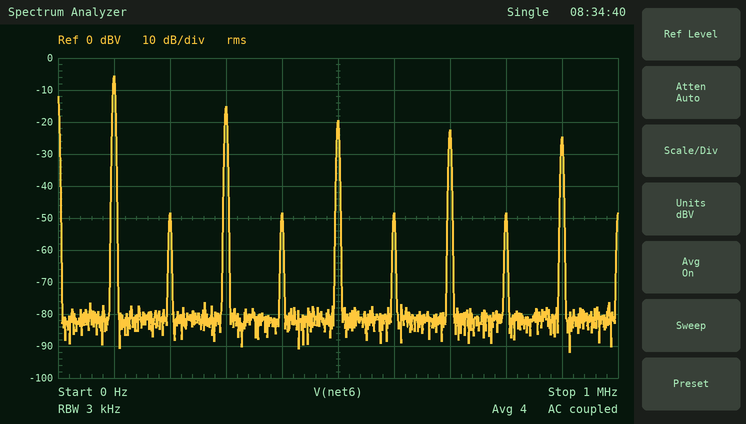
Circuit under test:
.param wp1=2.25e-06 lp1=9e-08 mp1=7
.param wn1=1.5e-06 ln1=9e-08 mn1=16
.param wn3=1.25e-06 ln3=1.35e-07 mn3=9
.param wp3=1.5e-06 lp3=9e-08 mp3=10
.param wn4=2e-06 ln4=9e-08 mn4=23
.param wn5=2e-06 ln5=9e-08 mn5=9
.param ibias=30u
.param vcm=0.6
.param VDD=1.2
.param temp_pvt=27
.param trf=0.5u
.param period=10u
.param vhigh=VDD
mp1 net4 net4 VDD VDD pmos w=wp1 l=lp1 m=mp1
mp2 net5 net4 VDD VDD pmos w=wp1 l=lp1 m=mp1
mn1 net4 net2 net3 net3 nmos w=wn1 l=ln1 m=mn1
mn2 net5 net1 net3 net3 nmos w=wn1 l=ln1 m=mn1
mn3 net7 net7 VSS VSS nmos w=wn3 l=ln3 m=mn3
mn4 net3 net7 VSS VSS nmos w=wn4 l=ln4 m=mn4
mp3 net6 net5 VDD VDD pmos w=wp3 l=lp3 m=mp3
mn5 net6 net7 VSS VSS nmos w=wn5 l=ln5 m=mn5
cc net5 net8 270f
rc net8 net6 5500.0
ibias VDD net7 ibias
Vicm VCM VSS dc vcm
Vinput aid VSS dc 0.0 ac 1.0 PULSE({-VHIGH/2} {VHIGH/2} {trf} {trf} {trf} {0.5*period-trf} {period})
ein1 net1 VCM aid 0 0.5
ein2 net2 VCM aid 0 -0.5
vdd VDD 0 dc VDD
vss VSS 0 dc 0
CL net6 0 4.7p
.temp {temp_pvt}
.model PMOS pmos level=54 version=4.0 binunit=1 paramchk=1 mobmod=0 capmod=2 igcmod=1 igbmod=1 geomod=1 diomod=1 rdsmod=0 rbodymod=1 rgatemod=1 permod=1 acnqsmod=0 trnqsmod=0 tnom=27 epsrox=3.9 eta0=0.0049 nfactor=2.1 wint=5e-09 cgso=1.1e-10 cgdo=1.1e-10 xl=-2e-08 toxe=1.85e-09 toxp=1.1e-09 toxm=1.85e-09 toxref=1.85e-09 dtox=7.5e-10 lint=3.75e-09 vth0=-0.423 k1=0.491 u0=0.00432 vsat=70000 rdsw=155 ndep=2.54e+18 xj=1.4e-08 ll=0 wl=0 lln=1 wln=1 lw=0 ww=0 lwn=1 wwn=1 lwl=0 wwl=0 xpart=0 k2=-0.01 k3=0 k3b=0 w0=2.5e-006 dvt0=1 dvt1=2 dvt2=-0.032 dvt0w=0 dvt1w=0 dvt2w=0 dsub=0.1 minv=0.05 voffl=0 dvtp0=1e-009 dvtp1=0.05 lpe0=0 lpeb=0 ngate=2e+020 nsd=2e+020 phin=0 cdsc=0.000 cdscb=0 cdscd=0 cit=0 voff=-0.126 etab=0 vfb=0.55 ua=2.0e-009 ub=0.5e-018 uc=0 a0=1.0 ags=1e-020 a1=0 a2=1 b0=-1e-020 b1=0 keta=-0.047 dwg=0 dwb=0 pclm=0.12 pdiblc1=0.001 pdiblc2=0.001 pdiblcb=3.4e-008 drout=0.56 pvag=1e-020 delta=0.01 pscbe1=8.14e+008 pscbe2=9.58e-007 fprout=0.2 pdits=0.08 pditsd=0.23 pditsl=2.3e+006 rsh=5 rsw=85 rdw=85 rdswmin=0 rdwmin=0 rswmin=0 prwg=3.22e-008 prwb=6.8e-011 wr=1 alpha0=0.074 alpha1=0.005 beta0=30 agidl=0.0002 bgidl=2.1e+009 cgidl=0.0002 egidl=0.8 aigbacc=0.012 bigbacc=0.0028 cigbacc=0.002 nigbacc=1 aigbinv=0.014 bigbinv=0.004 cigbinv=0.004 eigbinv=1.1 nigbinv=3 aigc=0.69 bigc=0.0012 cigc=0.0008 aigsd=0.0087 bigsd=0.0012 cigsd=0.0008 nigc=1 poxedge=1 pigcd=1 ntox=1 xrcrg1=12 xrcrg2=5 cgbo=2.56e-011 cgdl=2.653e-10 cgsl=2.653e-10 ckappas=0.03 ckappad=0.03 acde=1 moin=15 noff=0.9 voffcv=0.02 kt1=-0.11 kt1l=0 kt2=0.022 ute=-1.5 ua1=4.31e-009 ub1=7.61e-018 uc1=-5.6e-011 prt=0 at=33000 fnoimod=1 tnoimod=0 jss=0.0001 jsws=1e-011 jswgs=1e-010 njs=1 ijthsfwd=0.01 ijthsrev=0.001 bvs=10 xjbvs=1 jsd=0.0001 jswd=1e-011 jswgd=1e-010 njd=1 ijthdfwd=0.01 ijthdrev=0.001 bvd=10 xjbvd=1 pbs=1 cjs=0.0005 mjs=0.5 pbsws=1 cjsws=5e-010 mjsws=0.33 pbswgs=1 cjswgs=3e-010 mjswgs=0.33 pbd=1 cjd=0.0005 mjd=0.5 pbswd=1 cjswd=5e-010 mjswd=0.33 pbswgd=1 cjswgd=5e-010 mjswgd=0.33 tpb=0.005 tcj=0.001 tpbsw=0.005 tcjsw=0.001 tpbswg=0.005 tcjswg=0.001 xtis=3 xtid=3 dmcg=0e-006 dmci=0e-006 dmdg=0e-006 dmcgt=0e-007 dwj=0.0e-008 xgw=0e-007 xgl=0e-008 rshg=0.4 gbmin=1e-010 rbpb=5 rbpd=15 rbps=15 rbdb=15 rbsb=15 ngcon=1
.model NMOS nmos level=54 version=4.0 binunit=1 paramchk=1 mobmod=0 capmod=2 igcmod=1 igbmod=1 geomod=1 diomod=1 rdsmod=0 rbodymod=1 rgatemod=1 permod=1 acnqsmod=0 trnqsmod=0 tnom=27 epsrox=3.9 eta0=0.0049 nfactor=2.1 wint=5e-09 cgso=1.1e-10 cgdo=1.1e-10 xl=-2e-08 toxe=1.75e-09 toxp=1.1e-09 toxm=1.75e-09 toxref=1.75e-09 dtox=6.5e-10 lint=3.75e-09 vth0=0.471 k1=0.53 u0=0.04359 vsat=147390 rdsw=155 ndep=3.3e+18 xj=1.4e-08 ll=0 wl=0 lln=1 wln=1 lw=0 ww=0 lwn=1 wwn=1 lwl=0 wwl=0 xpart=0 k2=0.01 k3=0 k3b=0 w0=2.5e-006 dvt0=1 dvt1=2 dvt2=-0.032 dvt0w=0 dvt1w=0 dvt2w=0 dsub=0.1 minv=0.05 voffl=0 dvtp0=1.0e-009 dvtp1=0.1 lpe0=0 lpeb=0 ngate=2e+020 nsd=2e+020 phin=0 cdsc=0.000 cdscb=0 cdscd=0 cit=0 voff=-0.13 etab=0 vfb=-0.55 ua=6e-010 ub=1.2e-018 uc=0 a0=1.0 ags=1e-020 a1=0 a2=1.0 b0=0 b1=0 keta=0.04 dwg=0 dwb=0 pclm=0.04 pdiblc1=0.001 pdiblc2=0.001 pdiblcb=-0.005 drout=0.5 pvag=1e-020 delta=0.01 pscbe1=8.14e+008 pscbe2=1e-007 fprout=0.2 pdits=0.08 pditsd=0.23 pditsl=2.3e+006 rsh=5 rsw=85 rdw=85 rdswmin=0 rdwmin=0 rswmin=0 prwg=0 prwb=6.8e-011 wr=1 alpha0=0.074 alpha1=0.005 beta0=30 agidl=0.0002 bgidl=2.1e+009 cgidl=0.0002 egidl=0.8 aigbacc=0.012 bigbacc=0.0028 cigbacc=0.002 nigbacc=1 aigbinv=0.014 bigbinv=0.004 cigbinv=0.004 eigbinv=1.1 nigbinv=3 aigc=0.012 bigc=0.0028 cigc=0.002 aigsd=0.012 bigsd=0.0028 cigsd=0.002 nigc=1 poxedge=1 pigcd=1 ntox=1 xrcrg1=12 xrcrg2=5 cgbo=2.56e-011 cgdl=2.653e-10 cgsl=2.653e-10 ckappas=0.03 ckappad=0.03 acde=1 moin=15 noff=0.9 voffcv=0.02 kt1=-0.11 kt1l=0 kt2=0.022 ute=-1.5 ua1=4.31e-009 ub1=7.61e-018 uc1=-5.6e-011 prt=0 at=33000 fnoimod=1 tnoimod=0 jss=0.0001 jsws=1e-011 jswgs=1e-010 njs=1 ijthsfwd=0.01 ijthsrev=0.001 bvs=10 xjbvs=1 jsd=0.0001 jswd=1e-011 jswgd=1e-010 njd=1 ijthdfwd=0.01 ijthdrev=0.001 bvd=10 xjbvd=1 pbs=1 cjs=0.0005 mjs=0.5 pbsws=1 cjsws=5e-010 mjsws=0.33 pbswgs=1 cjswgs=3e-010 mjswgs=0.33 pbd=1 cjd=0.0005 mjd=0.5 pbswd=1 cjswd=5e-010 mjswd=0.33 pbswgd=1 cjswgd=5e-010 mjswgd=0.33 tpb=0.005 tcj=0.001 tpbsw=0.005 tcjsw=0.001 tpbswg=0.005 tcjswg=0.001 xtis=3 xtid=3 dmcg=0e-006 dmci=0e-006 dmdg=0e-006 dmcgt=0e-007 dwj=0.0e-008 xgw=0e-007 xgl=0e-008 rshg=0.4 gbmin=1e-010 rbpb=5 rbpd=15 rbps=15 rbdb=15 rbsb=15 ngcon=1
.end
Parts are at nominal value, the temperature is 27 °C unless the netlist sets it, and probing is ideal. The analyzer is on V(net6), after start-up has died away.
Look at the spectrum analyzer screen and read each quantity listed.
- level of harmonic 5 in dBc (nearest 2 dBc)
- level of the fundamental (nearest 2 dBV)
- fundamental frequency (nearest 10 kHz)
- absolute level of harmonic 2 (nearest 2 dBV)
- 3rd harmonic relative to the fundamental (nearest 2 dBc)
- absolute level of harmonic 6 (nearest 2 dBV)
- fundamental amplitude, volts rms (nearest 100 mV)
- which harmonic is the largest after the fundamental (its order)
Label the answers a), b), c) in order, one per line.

a) -14 dBc
b) -6 dBV
c) 100 kHz
d) -48 dBV
e) -10 dBc
f) -48 dBV
g) 500 mV
h) 3
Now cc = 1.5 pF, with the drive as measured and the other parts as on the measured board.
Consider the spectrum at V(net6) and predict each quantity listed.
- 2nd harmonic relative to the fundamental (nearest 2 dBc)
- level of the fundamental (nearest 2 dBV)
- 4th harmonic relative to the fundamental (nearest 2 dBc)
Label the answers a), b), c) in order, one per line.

a) -40 dBc
b) -6 dBV
c) -40 dBc
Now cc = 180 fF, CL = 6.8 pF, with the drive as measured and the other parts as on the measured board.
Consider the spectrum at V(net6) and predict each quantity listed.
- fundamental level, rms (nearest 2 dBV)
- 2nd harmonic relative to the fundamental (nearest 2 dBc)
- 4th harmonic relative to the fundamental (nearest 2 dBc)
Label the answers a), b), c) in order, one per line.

a) -6 dBV
b) -40 dBc
c) -40 dBc
